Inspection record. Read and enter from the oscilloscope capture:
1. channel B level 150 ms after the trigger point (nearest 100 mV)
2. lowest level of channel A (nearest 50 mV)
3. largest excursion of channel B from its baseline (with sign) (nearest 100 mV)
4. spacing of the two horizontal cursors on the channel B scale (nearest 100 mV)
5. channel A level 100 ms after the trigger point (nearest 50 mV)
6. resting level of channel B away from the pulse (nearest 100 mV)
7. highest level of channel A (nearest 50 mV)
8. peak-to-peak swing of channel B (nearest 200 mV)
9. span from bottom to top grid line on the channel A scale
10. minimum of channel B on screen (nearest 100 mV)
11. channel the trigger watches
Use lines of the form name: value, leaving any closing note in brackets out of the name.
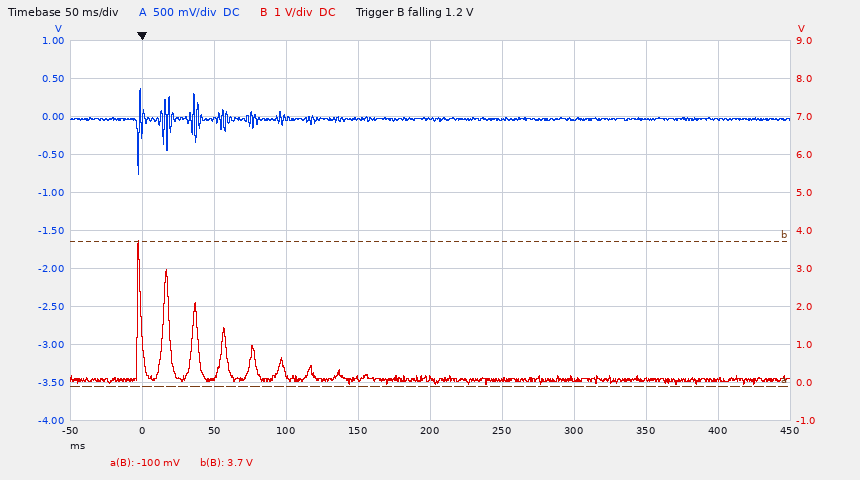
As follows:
channel B level 150 ms after the trigger point: 100 mV
lowest level of channel A: -750 mV
largest excursion of channel B from its baseline (with sign): +3.7 V
spacing of the two horizontal cursors on the channel B scale: 3.8 V
channel A level 100 ms after the trigger point: 0 mV
resting level of channel B away from the pulse: 100 mV
highest level of channel A: 350 mV
peak-to-peak swing of channel B: 3.8 V
span from bottom to top grid line on the channel A scale: 5 V
minimum of channel B on screen: -100 mV
channel the trigger watches: channel B
